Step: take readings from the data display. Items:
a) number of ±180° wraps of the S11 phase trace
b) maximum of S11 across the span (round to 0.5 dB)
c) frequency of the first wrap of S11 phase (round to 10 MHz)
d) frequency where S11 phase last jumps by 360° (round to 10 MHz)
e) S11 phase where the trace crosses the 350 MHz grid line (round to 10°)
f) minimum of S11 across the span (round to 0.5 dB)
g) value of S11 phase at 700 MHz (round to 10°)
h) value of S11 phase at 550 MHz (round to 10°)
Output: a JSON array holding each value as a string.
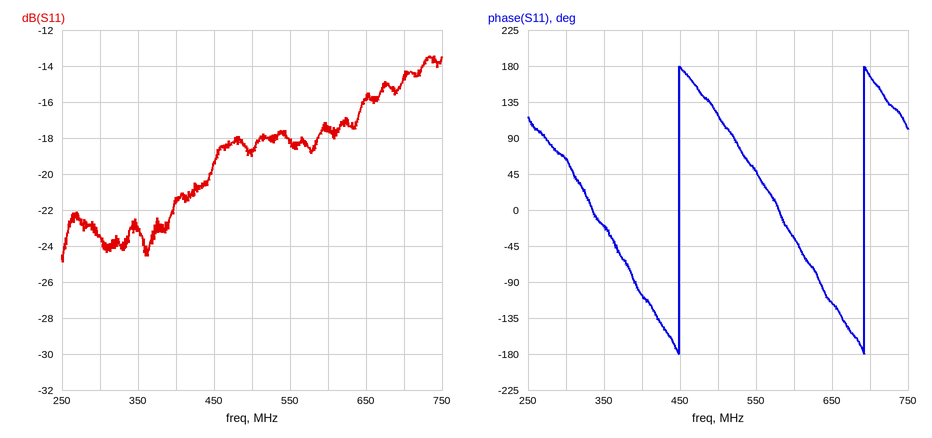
["2", "-13.5 dB", "450 MHz", "690 MHz", "-20°", "-25.0 dB", "170°", "50°"]
